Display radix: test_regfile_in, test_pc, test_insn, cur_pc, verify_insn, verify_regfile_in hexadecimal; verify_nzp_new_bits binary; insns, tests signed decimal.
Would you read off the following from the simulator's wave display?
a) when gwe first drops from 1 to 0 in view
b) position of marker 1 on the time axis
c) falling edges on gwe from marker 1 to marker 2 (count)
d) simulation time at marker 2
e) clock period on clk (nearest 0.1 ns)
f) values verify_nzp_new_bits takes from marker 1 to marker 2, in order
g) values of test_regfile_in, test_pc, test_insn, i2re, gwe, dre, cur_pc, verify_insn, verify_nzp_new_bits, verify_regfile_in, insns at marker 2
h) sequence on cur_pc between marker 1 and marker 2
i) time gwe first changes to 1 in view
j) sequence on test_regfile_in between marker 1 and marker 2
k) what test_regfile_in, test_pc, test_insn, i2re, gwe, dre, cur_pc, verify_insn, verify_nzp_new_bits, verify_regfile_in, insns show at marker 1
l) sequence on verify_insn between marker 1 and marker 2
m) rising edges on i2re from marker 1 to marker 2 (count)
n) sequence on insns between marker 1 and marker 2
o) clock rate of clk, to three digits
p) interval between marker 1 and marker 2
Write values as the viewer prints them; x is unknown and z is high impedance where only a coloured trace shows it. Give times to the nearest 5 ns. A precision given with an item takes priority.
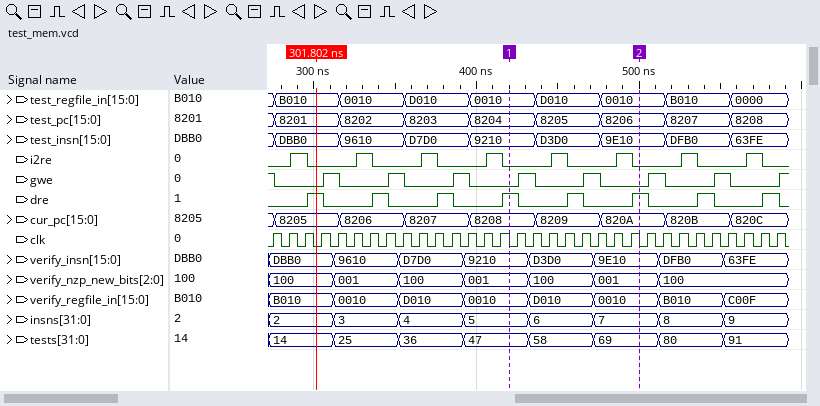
275 ns
420 ns
2
500 ns
10 ns
001, 100, 001
test_regfile_in=0010, test_pc=8206, test_insn=9E10, i2re=0, gwe=0, dre=1, cur_pc=820A, verify_insn=9E10, verify_nzp_new_bits=001, verify_regfile_in=0010, insns=7
8208, 8209, 820A
305 ns
0010, D010, 0010
test_regfile_in=0010, test_pc=8204, test_insn=9210, i2re=0, gwe=0, dre=1, cur_pc=8208, verify_insn=9210, verify_nzp_new_bits=001, verify_regfile_in=0010, insns=5
9210, D3D0, 9E10
2
5, 6, 7
100 MHz
80 ns
